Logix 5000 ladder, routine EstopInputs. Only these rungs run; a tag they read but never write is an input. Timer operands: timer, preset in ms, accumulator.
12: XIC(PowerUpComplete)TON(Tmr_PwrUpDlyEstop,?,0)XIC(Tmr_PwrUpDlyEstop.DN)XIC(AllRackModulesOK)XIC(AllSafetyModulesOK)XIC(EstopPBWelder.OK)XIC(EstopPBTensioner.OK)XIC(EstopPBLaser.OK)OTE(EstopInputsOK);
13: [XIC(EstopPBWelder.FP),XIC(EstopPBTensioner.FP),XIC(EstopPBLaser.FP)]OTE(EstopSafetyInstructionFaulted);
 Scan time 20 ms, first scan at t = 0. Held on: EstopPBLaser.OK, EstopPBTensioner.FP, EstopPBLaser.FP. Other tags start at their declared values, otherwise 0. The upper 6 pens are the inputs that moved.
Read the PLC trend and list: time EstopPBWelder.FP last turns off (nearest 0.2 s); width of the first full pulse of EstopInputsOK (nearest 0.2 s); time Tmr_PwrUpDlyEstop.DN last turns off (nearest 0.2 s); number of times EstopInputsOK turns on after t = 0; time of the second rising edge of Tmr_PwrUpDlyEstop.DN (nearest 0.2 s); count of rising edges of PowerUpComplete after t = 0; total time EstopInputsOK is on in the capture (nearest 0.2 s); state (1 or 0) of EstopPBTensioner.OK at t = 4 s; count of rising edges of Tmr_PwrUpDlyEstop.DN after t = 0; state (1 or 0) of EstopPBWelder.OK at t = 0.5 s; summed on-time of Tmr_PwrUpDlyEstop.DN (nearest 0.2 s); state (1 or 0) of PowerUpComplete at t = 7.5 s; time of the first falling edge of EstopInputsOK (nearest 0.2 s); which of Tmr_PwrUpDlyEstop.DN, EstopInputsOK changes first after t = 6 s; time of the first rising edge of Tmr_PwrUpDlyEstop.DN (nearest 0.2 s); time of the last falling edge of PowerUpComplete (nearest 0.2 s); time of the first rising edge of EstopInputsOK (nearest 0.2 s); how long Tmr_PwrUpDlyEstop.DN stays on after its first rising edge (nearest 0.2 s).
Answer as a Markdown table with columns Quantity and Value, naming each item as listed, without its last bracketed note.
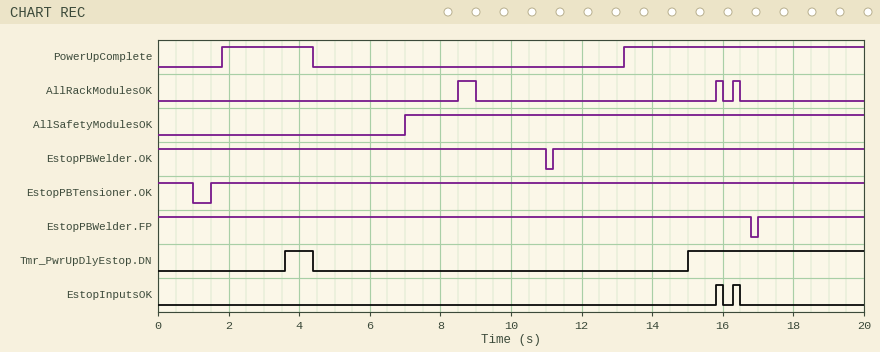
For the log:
| Quantity | Value |
|---|---|
| time EstopPBWelder.FP last turns off | 16.8 s |
| width of the first full pulse of EstopInputsOK | 0.2 s |
| time Tmr_PwrUpDlyEstop.DN last turns off | 4.4 s |
| number of times EstopInputsOK turns on after t = 0 | 2 |
| time of the second rising edge of Tmr_PwrUpDlyEstop.DN | 15.0 s |
| count of rising edges of PowerUpComplete after t = 0 | 2 |
| total time EstopInputsOK is on in the capture | 0.4 s |
| state (1 or 0) of EstopPBTensioner.OK at t = 4 s | 1 |
| count of rising edges of Tmr_PwrUpDlyEstop.DN after t = 0 | 2 |
| state (1 or 0) of EstopPBWelder.OK at t = 0.5 s | 1 |
| summed on-time of Tmr_PwrUpDlyEstop.DN | 5.8 s |
| state (1 or 0) of PowerUpComplete at t = 7.5 s | 0 |
| time of the first falling edge of EstopInputsOK | 16.0 s |
| which of Tmr_PwrUpDlyEstop.DN, EstopInputsOK changes first after t = 6 s | Tmr_PwrUpDlyEstop.DN |
| time of the first rising edge of Tmr_PwrUpDlyEstop.DN | 3.6 s |
| time of the last falling edge of PowerUpComplete | 4.4 s |
| time of the first rising edge of EstopInputsOK | 15.8 s |
| how long Tmr_PwrUpDlyEstop.DN stays on after its first rising edge | 0.8 s |
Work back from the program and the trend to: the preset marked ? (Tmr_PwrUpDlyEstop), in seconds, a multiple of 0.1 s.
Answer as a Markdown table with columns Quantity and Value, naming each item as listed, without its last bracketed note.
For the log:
| Quantity | Value |
|---|---|
| the preset marked ? (Tmr_PwrUpDlyEstop), in seconds, a multiple of 0.1 s | 1.8 s |
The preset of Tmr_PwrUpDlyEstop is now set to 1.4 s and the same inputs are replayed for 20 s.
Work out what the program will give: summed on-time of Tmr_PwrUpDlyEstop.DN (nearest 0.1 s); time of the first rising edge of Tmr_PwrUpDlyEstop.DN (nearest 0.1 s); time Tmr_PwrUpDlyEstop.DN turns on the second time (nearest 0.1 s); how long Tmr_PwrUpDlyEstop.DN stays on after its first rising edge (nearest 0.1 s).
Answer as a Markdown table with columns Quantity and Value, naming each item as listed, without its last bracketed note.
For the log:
| Quantity | Value |
|---|---|
| summed on-time of Tmr_PwrUpDlyEstop.DN | 6.6 s |
| time of the first rising edge of Tmr_PwrUpDlyEstop.DN | 3.2 s |
| time Tmr_PwrUpDlyEstop.DN turns on the second time | 14.6 s |
| how long Tmr_PwrUpDlyEstop.DN stays on after its first rising edge | 1.2 s |
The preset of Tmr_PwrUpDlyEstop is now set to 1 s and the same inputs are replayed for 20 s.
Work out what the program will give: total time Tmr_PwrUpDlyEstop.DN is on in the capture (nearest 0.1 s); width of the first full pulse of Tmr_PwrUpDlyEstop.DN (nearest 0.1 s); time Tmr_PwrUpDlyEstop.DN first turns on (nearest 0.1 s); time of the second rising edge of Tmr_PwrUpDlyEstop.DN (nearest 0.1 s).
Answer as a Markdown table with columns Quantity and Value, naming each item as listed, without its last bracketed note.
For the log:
| Quantity | Value |
|---|---|
| total time Tmr_PwrUpDlyEstop.DN is on in the capture | 7.4 s |
| width of the first full pulse of Tmr_PwrUpDlyEstop.DN | 1.6 s |
| time Tmr_PwrUpDlyEstop.DN first turns on | 2.8 s |
| time of the second rising edge of Tmr_PwrUpDlyEstop.DN | 14.2 s |
